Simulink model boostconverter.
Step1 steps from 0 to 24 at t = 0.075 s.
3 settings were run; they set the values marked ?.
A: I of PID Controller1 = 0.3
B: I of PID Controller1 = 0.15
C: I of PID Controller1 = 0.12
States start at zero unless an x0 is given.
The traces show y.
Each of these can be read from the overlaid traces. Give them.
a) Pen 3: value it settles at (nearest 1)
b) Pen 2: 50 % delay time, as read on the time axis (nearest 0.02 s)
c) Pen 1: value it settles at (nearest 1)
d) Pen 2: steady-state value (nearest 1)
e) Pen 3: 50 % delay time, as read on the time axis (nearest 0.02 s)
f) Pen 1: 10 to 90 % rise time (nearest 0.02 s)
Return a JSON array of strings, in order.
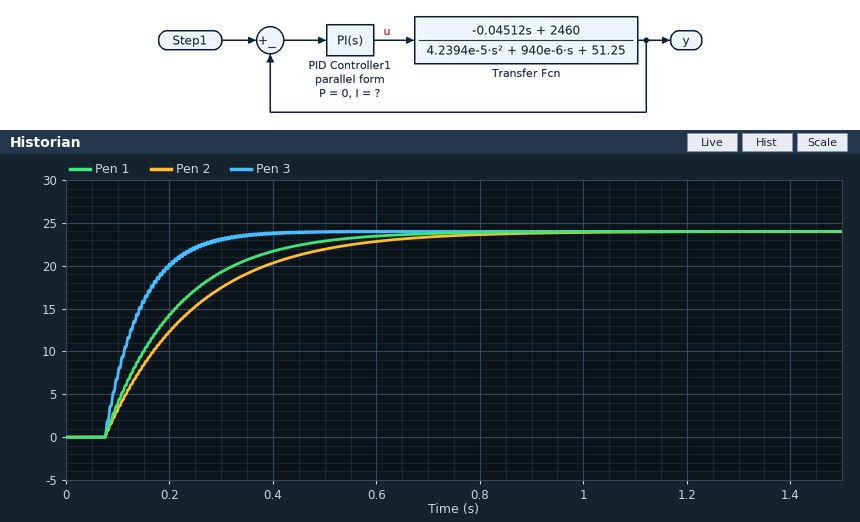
["24", "0.20 s", "24", "24", "0.12 s", "0.30 s"]
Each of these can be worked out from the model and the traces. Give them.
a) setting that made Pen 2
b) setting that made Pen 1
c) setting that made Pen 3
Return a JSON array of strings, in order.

["C", "B", "A"]
